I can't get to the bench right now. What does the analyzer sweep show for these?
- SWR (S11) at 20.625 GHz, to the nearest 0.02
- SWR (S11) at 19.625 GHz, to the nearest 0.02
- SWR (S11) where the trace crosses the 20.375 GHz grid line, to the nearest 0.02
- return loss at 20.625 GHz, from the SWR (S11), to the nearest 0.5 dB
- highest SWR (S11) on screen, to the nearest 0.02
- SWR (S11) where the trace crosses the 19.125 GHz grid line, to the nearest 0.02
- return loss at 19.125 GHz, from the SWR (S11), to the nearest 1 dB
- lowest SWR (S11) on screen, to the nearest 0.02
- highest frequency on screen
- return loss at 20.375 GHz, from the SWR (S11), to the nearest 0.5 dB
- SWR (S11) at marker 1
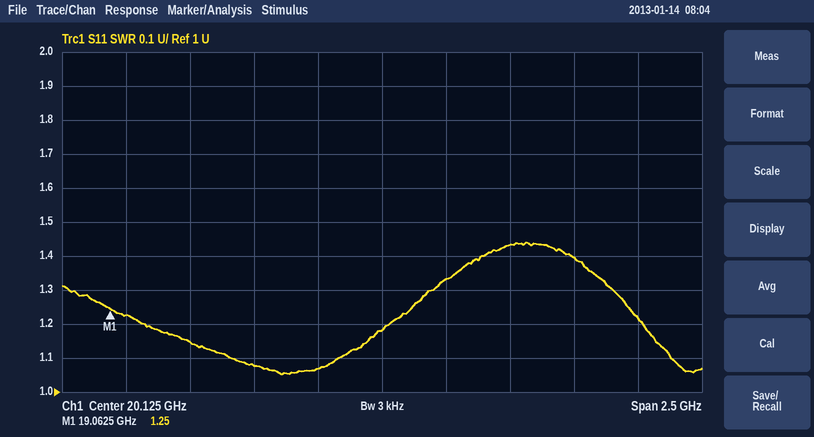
1.44
1.08
1.34
15.0 dB
1.44
1.22
20 dB
1.06
21.375 GHz
17.0 dB
1.25
